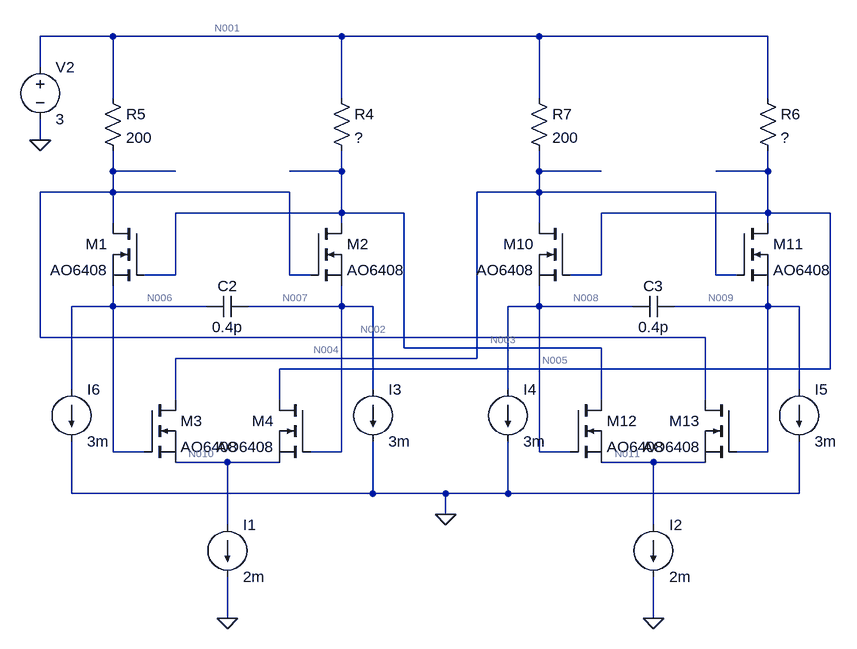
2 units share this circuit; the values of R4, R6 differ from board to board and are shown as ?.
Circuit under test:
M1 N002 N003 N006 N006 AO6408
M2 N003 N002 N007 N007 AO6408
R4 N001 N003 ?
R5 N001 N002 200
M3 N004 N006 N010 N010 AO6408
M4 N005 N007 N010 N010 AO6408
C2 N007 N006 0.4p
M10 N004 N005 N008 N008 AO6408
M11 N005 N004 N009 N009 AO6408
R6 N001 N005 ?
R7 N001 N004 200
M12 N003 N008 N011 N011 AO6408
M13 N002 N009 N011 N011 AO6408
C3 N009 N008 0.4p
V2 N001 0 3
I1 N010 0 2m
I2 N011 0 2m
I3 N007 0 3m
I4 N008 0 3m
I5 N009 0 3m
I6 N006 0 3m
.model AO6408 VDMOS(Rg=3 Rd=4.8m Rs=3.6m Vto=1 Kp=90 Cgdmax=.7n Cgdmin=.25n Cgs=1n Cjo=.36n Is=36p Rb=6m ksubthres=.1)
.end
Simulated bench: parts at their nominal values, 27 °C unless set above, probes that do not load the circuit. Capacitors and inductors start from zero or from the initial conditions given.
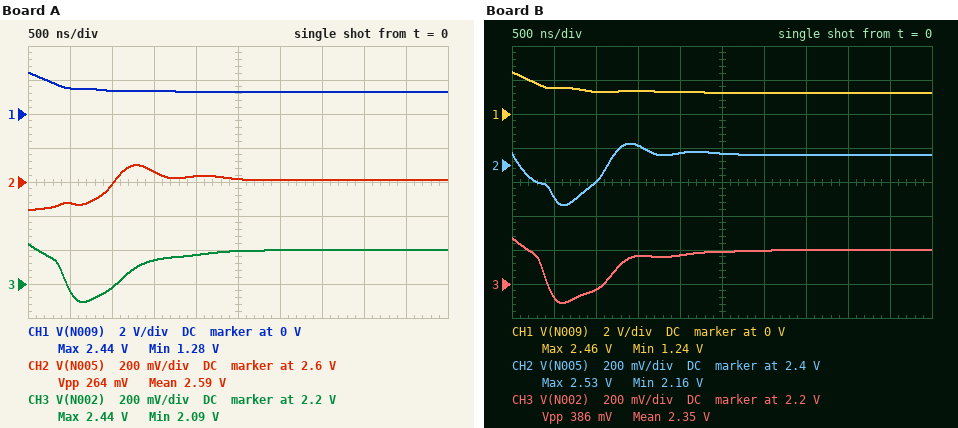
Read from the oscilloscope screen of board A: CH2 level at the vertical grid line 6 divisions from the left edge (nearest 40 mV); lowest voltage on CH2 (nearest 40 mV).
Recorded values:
2.60 V
2.44 V
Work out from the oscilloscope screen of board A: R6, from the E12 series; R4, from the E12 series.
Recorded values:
120 Ω
100 Ω
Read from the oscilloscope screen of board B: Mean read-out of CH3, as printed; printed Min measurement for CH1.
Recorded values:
2.35 V
1.24 V
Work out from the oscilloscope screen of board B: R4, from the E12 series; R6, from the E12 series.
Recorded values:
68 Ω
180 Ω
